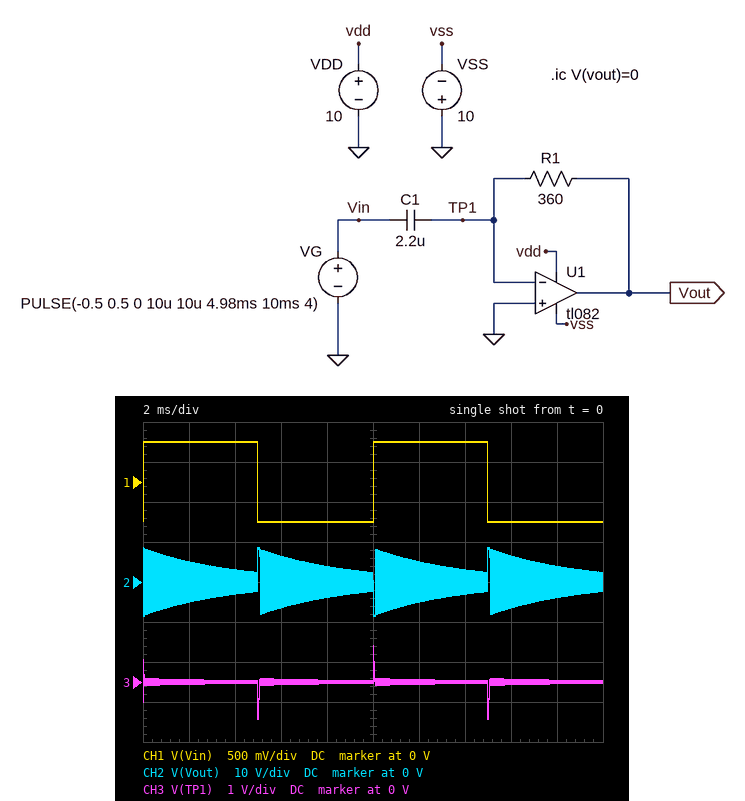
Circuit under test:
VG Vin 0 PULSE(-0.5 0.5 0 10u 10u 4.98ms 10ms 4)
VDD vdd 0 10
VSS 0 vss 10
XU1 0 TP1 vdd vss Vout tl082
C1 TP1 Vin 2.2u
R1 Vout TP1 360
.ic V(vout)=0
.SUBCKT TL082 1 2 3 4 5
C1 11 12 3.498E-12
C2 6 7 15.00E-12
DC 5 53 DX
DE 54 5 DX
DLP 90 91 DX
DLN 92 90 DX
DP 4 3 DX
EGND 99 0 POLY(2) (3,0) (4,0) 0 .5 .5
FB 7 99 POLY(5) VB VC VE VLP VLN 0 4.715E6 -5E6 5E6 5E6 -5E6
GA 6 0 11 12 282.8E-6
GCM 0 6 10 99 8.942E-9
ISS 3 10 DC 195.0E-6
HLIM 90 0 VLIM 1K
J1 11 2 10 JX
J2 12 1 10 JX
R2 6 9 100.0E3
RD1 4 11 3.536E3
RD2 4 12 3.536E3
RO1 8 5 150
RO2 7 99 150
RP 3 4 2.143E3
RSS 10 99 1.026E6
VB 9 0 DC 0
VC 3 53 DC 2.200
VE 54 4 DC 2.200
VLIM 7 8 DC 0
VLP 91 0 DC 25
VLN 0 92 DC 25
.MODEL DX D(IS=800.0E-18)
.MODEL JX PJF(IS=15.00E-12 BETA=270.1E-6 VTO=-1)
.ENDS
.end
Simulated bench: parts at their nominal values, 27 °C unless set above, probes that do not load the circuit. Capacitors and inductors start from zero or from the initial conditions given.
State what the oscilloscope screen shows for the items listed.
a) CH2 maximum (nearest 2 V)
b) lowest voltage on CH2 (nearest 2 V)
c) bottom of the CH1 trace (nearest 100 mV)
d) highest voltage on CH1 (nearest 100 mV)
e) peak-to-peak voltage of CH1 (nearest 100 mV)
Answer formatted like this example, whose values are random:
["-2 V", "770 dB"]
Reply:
["8 V", "-8 V", "-500 mV", "500 mV", "1.0 V"]
